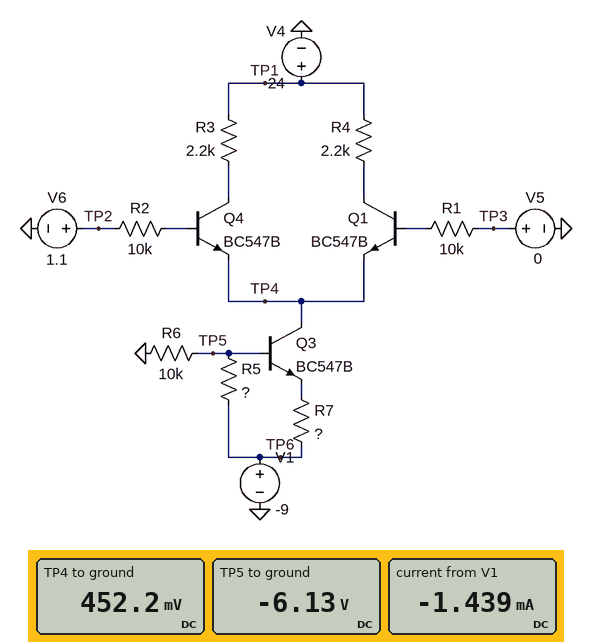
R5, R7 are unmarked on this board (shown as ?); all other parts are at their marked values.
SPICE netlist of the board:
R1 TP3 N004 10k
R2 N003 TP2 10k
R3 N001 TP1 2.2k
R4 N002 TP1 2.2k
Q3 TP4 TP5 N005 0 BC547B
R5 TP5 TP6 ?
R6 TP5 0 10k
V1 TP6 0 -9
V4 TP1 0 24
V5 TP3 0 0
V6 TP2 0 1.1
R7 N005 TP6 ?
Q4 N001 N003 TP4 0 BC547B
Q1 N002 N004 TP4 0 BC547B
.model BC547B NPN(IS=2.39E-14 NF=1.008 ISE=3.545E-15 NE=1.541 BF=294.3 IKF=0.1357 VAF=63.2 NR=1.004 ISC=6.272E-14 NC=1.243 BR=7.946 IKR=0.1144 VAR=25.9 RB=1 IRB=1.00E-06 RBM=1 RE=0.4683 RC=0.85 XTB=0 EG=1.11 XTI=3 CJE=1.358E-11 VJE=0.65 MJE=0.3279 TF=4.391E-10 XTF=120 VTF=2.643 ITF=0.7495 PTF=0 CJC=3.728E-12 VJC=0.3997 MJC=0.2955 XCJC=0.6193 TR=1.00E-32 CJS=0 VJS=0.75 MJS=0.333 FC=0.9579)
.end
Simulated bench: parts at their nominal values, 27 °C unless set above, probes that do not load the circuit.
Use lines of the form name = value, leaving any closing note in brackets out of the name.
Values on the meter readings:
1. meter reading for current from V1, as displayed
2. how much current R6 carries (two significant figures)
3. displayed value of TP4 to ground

meter reading for current from V1, as displayed = -1.439 mA
how much current R6 carries = 610 µA
displayed value of TP4 to ground = 452.2 mV
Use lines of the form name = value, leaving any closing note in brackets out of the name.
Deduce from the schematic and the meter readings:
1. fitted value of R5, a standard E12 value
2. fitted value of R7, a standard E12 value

fitted value of R5, a standard E12 value = 4.7 kΩ
fitted value of R7, a standard E12 value = 2.7 kΩ
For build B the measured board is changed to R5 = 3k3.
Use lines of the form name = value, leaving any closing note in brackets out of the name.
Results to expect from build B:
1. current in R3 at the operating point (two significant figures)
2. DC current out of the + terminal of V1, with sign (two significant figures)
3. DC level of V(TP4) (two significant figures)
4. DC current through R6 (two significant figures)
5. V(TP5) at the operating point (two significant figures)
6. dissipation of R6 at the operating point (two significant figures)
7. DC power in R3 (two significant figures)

current in R3 at the operating point = 590 µA
DC current out of the + terminal of V1, with sign = -1.3 mA
DC level of V(TP4) = 470 mV
DC current through R6 = 680 µA
V(TP5) at the operating point = -6.8 V
dissipation of R6 at the operating point = 4.6 mW
DC power in R3 = 770 µW
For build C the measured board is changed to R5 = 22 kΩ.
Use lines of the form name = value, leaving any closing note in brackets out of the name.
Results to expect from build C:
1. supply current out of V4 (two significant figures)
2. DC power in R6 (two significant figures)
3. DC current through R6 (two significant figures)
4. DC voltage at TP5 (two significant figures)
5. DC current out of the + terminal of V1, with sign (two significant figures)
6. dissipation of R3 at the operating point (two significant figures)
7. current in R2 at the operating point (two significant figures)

supply current out of V4 = 2.0 mA
DC power in R6 = 820 µW
DC current through R6 = 290 µA
DC voltage at TP5 = -2.9 V
DC current out of the + terminal of V1, with sign = -2.3 mA
dissipation of R3 at the operating point = 9.0 mW
current in R2 at the operating point = 5.5 µA
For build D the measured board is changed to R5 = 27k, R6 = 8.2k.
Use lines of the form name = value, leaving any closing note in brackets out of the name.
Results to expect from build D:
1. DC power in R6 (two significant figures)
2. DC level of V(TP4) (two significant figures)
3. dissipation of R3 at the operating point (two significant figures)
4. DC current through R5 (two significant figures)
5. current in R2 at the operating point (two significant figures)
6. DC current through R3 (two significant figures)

DC power in R6 = 560 µW
DC level of V(TP4) = 380 mV
dissipation of R3 at the operating point = 11 mW
DC current through R5 = 250 µA
current in R2 at the operating point = 6.3 µA
DC current through R3 = 2.3 mA
